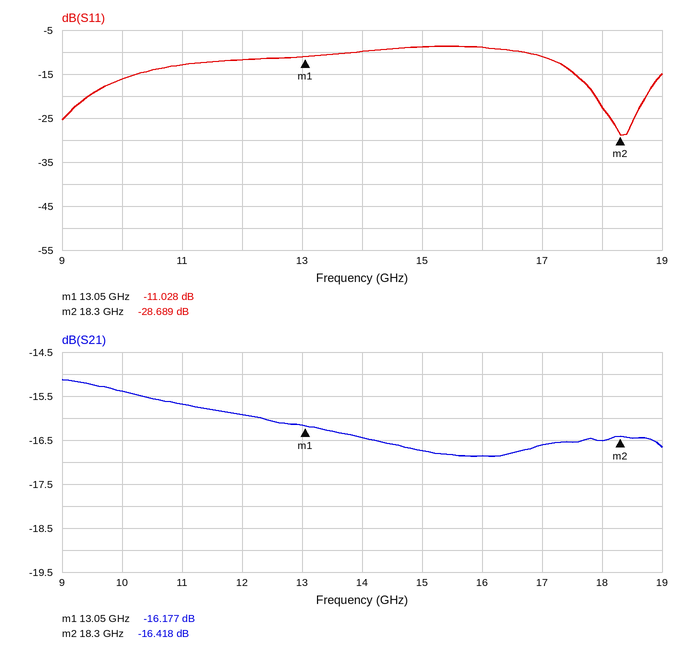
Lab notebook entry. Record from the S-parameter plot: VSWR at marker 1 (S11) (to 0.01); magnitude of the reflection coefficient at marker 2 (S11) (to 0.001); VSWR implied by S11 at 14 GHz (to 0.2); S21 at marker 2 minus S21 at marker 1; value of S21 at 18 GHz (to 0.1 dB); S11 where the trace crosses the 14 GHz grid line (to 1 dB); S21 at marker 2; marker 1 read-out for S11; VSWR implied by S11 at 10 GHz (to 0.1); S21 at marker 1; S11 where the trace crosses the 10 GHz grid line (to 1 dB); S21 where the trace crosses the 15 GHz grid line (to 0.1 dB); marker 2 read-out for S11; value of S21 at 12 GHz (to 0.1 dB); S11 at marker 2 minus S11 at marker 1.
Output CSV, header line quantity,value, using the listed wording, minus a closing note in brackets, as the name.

quantity,value
VSWR at marker 1 (S11),1.78
magnitude of the reflection coefficient at marker 2 (S11),0.037
VSWR implied by S11 at 14 GHz,2.0
S21 at marker 2 minus S21 at marker 1,-0.241 dB
value of S21 at 18 GHz,-16.5 dB
S11 where the trace crosses the 14 GHz grid line,-10 dB
S21 at marker 2,-16.418 dB
marker 1 read-out for S11,-11.028 dB
VSWR implied by S11 at 10 GHz,1.4
S21 at marker 1,-16.177 dB
S11 where the trace crosses the 10 GHz grid line,-16 dB
S21 where the trace crosses the 15 GHz grid line,-16.7 dB
marker 2 read-out for S11,-28.689 dB
value of S21 at 12 GHz,-15.9 dB
S11 at marker 2 minus S11 at marker 1,-17.661 dB
